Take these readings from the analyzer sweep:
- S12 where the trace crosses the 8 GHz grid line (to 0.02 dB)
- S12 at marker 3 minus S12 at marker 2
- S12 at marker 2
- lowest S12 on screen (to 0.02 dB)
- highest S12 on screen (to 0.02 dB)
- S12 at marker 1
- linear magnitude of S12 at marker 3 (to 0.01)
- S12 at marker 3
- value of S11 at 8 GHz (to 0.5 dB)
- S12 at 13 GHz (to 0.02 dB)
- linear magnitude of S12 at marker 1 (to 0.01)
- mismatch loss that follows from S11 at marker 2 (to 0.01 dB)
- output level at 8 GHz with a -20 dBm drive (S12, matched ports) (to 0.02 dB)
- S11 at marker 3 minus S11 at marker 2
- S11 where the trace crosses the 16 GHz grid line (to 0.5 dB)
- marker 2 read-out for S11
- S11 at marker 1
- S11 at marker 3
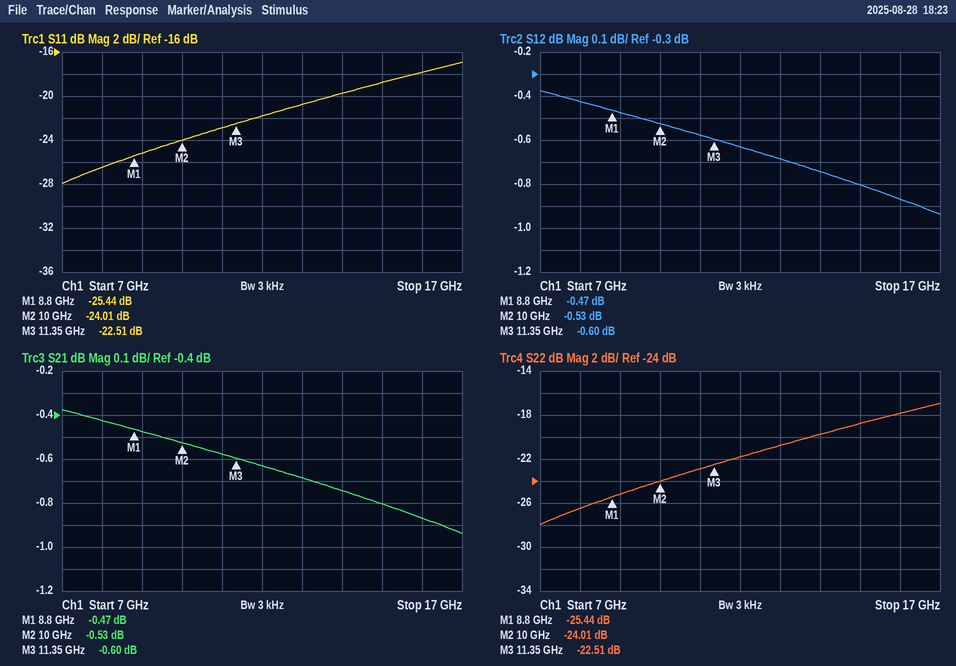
-0.42 dB
-0.07 dB
-0.53 dB
-0.94 dB
-0.38 dB
-0.47 dB
0.93
-0.60 dB
-26.5 dB
-0.68 dB
0.95
0.02 dB
-20.42 dBm
1.50 dB
-18.0 dB
-24.01 dB
-25.44 dB
-22.51 dB
